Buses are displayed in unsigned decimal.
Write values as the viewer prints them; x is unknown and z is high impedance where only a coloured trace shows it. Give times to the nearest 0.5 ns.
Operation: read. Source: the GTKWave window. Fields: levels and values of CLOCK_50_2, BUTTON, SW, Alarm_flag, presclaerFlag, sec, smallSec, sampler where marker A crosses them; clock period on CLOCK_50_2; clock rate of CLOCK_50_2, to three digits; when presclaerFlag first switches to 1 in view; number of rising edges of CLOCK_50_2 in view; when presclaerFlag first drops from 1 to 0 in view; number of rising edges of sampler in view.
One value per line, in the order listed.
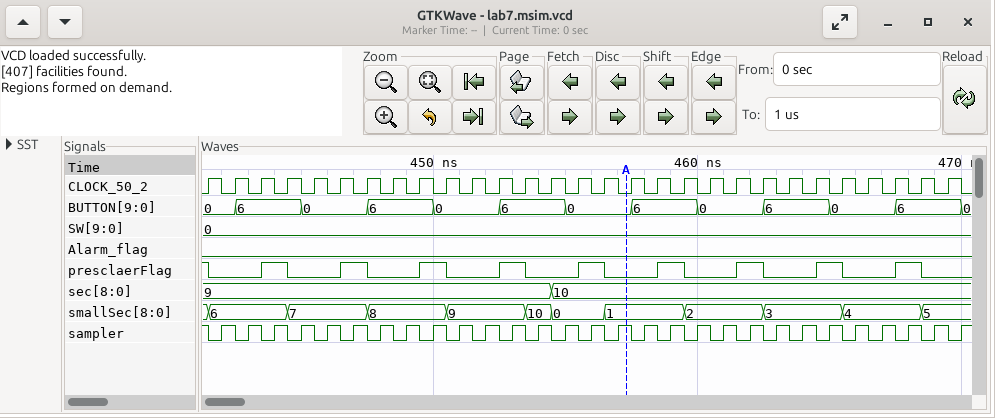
CLOCK_50_2=0, BUTTON=0, SW=0, Alarm_flag=0, presclaerFlag=0, sec=10, smallSec=1, sampler=1
1 ns
1.00 GHz
443.5 ns
29
441.5 ns
29
